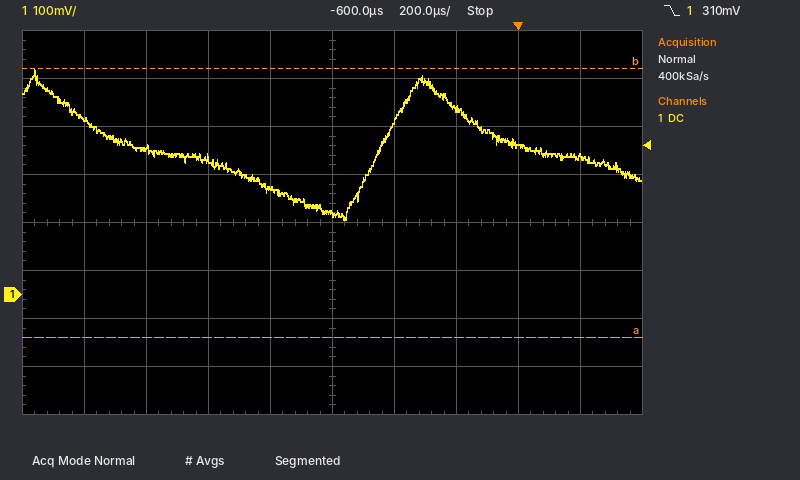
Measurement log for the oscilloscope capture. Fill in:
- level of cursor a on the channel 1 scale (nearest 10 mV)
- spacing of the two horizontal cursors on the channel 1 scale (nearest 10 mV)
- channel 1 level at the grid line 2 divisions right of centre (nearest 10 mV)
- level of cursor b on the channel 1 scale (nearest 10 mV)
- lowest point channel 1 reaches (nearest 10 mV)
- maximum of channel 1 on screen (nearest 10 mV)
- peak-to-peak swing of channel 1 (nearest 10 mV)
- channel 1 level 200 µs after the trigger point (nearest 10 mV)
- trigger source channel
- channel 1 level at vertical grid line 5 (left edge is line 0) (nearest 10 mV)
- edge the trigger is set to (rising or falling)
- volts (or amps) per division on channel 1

-90 mV
560 mV
390 mV
470 mV
160 mV
470 mV
310 mV
290 mV
channel 1
170 mV
falling
100 mV
